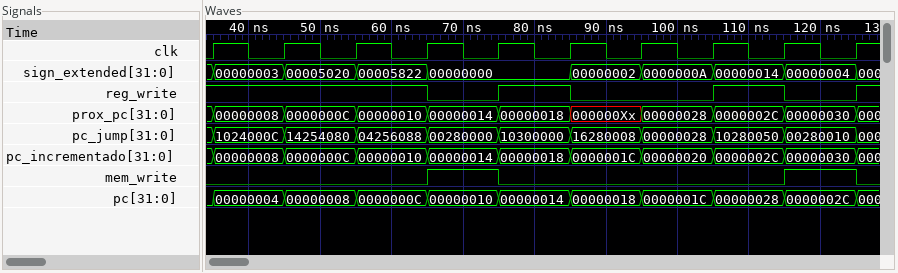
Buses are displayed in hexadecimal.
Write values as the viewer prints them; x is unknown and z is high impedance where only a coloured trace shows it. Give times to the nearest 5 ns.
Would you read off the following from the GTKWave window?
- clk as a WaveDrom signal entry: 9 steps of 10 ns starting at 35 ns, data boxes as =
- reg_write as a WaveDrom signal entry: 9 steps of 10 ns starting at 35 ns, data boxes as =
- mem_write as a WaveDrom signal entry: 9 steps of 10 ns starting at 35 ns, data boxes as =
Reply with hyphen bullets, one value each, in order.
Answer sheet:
- {name: 'clk', wave: 'p........'}
- {name: 'reg_write', wave: '1..010.10'}
- {name: 'mem_write', wave: '0..10...1'}
